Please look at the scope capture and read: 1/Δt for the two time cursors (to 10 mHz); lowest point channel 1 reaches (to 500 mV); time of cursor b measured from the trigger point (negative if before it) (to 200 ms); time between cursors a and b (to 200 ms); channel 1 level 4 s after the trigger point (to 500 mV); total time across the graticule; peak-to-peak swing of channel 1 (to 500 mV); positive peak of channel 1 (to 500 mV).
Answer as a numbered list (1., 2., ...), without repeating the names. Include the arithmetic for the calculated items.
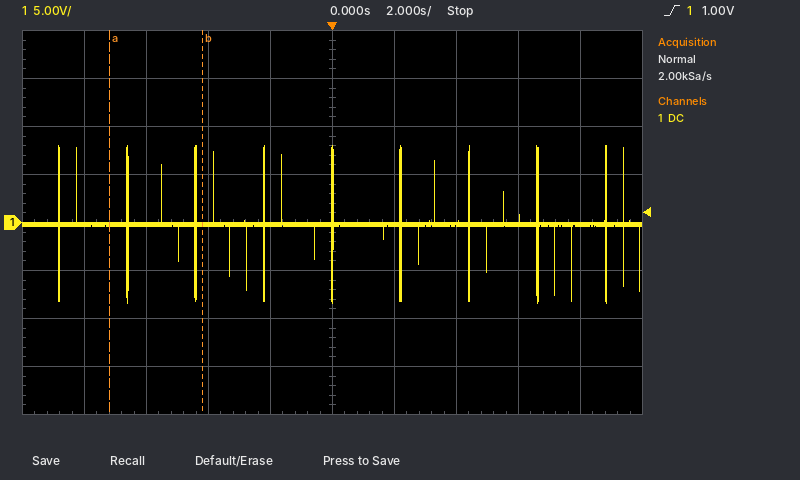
1. 1 / 3.0 s ≈ 330 mHz
2. -8.5 V
3. -4.2 s
4. 3.0 s
5. 0.0 V
6. 20 s
7. 8.0 V − (-8.5 V) = 16.5 V
8. 8.0 V
